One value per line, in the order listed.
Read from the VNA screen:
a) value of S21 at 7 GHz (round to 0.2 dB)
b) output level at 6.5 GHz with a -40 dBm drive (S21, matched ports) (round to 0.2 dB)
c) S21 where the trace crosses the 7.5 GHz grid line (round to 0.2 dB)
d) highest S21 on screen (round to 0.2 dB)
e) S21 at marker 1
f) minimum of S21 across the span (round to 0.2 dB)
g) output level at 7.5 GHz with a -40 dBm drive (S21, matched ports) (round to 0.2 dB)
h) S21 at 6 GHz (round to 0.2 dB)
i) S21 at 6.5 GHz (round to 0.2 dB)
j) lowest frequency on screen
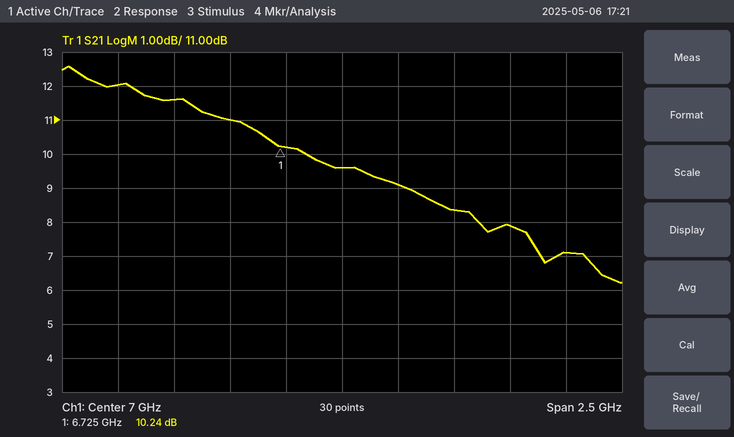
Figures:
9.6 dB
-29.0 dBm
8.4 dB
12.6 dB
10.24 dB
6.2 dB
-31.6 dBm
12.0 dB
11.0 dB
5.75 GHz
